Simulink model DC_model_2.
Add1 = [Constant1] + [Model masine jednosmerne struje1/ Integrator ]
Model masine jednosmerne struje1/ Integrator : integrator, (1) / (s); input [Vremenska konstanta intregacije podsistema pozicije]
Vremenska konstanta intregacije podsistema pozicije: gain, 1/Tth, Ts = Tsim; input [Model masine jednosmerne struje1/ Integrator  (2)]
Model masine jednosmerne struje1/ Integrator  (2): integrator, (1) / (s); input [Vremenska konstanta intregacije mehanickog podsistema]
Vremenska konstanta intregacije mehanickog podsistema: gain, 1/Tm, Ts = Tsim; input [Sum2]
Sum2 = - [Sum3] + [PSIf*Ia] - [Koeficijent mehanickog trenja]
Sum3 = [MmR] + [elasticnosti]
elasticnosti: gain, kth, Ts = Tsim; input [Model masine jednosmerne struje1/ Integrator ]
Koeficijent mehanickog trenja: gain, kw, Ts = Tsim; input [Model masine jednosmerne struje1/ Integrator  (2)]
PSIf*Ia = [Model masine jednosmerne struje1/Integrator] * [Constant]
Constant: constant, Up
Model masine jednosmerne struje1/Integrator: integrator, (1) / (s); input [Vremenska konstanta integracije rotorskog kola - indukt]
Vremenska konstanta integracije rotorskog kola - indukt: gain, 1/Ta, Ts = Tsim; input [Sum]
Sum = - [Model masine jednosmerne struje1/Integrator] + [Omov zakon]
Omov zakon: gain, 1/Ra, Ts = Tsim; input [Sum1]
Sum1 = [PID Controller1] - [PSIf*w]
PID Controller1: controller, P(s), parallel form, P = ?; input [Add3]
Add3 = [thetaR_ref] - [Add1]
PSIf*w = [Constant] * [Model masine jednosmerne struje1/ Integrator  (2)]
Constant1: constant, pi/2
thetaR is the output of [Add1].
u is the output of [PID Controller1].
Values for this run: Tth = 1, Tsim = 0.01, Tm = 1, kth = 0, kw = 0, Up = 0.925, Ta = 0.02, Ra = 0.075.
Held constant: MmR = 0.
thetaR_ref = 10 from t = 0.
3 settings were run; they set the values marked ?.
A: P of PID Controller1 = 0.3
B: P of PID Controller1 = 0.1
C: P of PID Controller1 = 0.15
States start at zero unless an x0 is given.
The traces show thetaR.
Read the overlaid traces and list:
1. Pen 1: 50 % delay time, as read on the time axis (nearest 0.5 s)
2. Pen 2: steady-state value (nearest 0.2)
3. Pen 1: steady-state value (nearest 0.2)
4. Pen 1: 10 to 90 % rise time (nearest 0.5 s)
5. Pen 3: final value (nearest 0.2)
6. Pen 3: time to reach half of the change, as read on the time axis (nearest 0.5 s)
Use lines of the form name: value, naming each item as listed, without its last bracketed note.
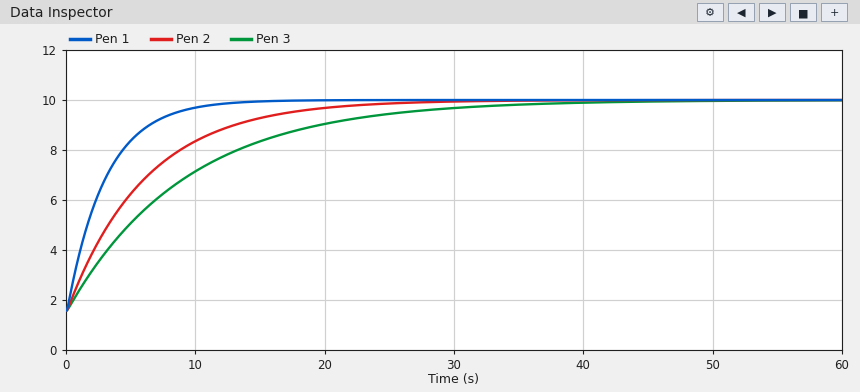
Pen 1: 50 % delay time, as read on the time axis: 2.0 s
Pen 2: steady-state value: 10.0
Pen 1: steady-state value: 10.0
Pen 1: 10 to 90 % rise time: 6.5 s
Pen 3: final value: 10.0
Pen 3: time to reach half of the change, as read on the time axis: 6.5 s
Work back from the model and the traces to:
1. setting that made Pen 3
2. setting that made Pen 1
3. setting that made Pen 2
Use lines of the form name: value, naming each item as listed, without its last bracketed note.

setting that made Pen 3: B
setting that made Pen 1: A
setting that made Pen 2: C
